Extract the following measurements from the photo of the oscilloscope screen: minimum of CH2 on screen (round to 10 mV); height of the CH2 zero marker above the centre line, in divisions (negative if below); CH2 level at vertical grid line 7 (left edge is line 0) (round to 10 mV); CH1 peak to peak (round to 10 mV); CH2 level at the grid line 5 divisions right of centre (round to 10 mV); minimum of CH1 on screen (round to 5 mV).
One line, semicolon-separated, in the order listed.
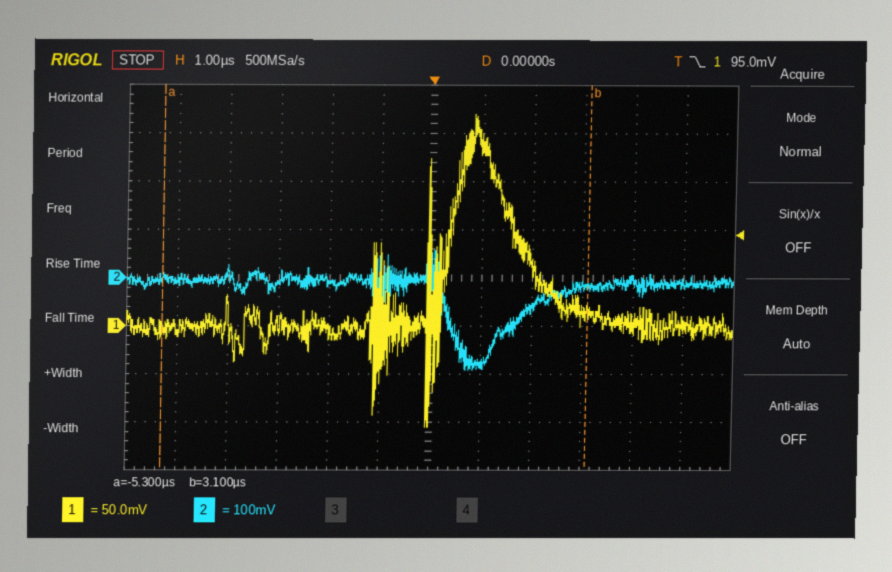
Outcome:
-190 mV; 0.0 div; -180 mV; 320 mV; -10 mV; -105 mV
